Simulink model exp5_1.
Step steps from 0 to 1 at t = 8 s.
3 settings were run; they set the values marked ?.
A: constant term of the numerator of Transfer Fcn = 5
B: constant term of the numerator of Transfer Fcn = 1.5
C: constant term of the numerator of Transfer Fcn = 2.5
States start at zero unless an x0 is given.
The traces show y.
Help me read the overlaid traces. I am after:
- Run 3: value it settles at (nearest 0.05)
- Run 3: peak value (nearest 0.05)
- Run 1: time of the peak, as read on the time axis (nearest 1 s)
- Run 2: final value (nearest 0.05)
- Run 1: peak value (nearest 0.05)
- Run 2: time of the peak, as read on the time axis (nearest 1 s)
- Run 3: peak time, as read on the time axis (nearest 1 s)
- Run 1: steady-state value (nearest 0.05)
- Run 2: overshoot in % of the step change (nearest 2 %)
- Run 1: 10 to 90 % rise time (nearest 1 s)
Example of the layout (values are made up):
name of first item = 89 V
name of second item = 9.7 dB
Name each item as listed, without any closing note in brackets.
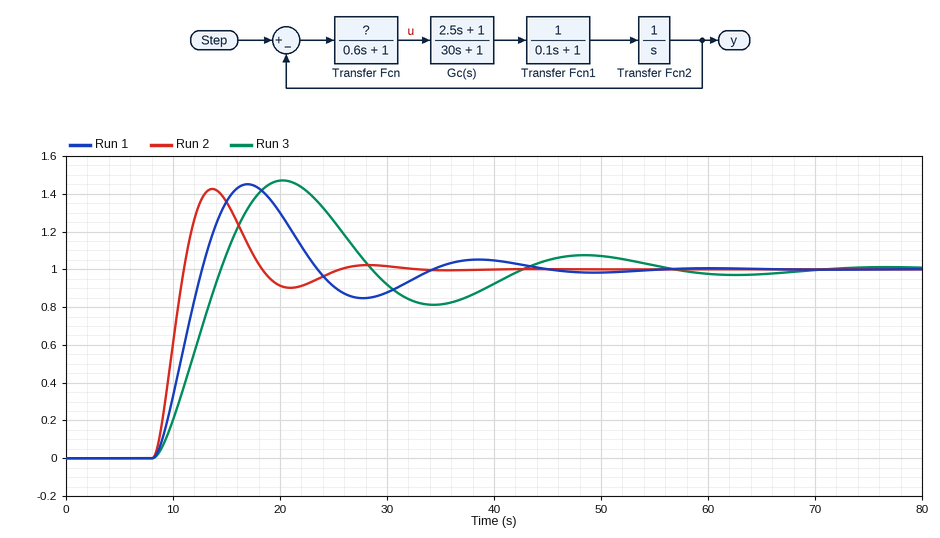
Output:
Run 3: value it settles at = 1.00
Run 3: peak value = 1.45
Run 1: time of the peak, as read on the time axis = 17 s
Run 2: final value = 1.00
Run 1: peak value = 1.45
Run 2: time of the peak, as read on the time axis = 14 s
Run 3: peak time, as read on the time axis = 20 s
Run 1: steady-state value = 1.00
Run 2: overshoot in % of the step change = 42 %
Run 1: 10 to 90 % rise time = 3 s
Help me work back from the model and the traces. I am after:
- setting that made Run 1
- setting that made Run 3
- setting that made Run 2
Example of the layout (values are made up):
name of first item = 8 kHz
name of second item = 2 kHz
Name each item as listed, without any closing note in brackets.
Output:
setting that made Run 1 = C
setting that made Run 3 = B
setting that made Run 2 = A
